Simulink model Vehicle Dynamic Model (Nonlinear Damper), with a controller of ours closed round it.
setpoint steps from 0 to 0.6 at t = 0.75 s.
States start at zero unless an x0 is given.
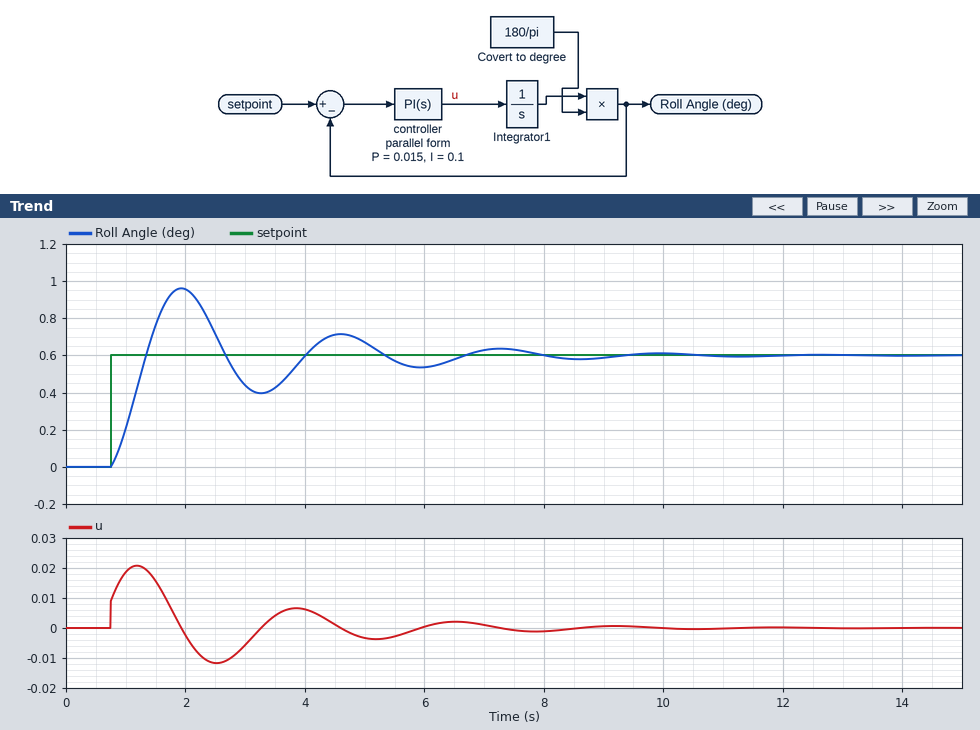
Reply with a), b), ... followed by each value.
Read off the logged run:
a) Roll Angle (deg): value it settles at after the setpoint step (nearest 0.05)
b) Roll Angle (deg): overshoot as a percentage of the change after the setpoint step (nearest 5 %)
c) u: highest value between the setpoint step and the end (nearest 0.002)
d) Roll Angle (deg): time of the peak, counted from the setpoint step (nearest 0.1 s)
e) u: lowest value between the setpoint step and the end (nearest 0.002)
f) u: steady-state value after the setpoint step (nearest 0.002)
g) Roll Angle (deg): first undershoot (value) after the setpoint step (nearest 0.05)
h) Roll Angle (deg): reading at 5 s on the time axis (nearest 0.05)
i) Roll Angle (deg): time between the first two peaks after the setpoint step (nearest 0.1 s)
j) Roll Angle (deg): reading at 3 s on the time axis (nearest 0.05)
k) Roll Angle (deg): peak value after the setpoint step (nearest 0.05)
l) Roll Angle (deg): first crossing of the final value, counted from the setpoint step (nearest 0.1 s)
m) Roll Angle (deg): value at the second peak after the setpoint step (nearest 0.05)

a) 0.60
b) 60 %
c) 0.020
d) 1.2 s
e) -0.012
f) 0.000
g) 0.40
h) 0.65
i) 2.7 s
j) 0.45
k) 0.95
l) 0.6 s
m) 0.70
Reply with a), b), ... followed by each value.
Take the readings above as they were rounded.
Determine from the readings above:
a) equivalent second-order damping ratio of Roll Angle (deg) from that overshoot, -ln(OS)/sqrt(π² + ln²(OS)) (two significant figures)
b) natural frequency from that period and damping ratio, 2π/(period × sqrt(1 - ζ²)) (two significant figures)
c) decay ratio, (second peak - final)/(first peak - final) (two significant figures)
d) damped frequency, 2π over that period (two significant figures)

a) 0.16
b) 2.4 rad/s
c) 0.29
d) 2.3 rad/s
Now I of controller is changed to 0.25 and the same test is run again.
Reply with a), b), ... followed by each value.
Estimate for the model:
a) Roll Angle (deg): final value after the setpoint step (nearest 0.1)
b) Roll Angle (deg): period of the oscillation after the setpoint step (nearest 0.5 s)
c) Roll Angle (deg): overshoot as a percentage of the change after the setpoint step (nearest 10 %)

a) 0.6
b) 1.5 s
c) 70 %
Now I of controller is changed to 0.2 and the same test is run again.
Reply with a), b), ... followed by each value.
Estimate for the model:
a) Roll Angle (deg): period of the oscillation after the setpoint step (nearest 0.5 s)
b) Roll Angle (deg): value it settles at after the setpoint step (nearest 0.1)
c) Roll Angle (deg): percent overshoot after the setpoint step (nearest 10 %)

a) 2.0 s
b) 0.6
c) 70 %
